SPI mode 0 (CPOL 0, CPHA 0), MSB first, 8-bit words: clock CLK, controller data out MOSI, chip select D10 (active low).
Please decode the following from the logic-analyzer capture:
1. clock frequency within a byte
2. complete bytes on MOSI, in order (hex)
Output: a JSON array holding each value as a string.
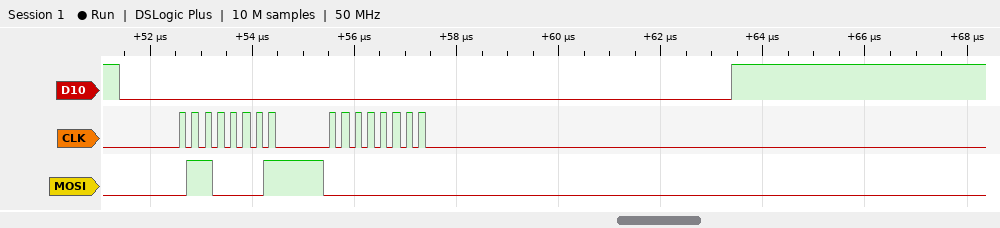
["4 MHz", "61 00"]
